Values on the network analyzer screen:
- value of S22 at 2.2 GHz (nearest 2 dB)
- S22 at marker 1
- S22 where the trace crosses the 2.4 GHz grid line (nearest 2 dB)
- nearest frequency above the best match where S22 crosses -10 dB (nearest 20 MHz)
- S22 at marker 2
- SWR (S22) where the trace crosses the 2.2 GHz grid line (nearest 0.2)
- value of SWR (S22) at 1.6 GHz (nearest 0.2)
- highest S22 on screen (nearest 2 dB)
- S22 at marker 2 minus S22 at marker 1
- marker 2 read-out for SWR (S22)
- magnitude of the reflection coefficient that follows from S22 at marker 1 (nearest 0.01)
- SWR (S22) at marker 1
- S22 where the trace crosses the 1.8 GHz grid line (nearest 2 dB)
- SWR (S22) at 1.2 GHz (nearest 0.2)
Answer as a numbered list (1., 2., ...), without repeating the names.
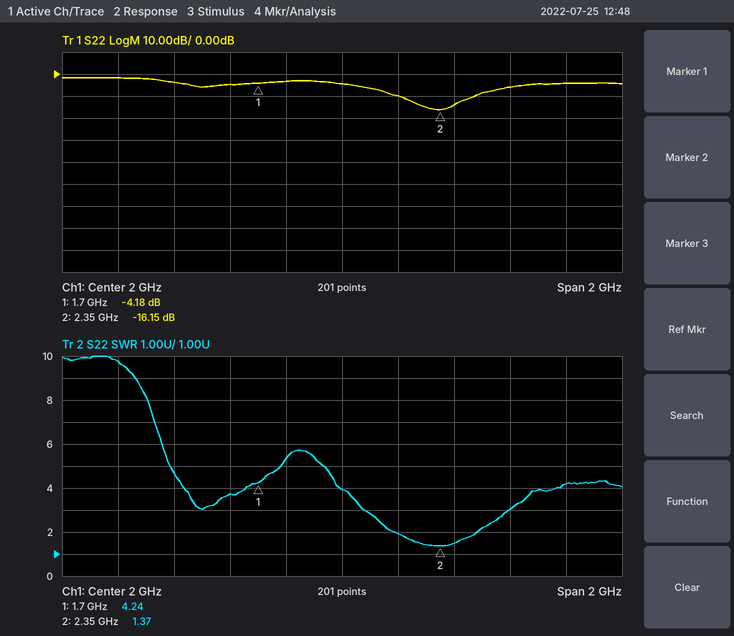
1. -10 dB
2. -4.18 dB
3. -14 dB
4. 2.48 GHz
5. -16.15 dB
6. 2.0
7. 3.8
8. -2 dB
9. -11.97 dB
10. 1.37
11. 0.62
12. 4.24
13. -4 dB
14. 9.8
